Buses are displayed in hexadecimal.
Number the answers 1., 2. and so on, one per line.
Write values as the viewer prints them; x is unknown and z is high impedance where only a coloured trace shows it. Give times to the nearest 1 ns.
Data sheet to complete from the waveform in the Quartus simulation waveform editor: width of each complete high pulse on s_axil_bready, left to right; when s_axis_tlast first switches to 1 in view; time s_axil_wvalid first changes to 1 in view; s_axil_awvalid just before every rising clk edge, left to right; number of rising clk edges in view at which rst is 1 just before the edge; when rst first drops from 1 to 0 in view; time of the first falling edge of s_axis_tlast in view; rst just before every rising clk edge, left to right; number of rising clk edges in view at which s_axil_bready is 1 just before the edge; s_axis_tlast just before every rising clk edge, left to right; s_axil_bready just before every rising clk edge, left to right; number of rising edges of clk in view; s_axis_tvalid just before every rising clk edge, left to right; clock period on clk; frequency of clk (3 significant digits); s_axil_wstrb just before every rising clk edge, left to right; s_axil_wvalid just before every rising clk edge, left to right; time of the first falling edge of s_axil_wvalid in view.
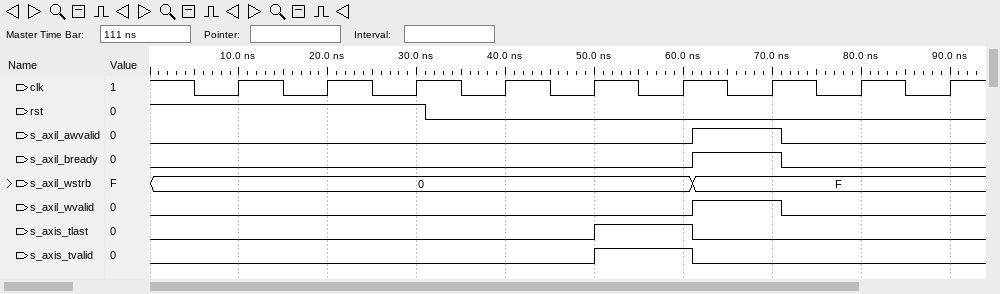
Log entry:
1. 10 ns
2. 50 ns
3. 61 ns
4. 0 0 0 0 0 0 1 0 0
5. 3
6. 31 ns
7. 61 ns
8. 1 1 1 0 0 0 0 0 0
9. 1
10. 0 0 0 0 0 1 0 0 0
11. 0 0 0 0 0 0 1 0 0
12. 9
13. 0 0 0 0 0 1 0 0 0
14. 10 ns
15. 100 MHz
16. 0, 0, 0, 0, 0, 0, F, F, F
17. 0 0 0 0 0 0 1 0 0
18. 71 ns
